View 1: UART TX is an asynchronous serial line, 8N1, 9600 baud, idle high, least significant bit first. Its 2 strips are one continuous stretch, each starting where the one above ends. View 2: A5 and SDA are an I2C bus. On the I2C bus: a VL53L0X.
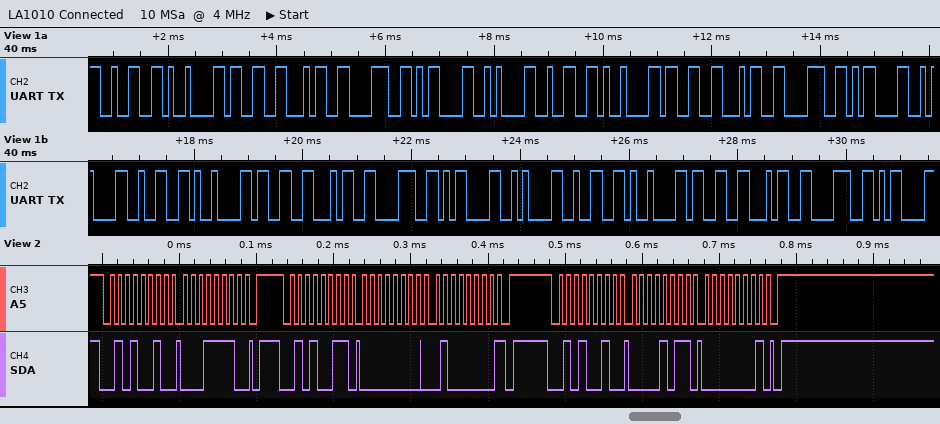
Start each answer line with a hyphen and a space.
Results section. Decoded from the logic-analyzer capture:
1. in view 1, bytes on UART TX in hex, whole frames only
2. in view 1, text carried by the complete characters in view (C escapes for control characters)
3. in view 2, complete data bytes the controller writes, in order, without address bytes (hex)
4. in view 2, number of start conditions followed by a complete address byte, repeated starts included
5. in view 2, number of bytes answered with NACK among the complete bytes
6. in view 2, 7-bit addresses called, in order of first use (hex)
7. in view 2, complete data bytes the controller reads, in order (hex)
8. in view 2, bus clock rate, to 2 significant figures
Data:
- 32 09 33 34 38 0D 0A 32 09 33 34 38 0D 0A 32 09 33 34 38 0D 0A 32 09 33 34 38 0D
- "2\t348\r\n2\t348\r\n2\t348\r\n2\t348\r"
- 1E 0B 01
- 3
- 1
- 0x29
- 00 40
- 100 kHz
